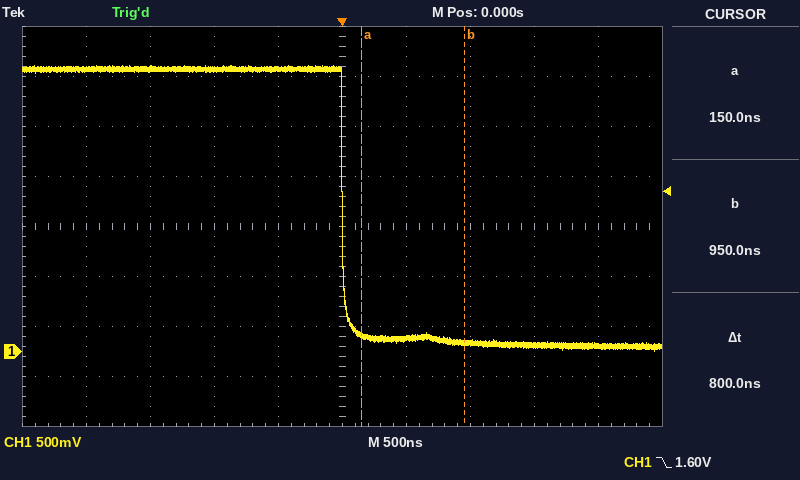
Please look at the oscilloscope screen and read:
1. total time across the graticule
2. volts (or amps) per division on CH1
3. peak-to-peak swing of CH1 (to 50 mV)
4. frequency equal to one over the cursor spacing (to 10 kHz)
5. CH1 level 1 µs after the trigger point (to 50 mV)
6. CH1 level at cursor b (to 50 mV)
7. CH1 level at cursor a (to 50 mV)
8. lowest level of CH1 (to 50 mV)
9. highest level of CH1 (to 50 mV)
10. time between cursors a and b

5 µs
500 mV
2.85 V
1.25 MHz
100 mV
100 mV
150 mV
0 mV
2.85 V
800 ns
